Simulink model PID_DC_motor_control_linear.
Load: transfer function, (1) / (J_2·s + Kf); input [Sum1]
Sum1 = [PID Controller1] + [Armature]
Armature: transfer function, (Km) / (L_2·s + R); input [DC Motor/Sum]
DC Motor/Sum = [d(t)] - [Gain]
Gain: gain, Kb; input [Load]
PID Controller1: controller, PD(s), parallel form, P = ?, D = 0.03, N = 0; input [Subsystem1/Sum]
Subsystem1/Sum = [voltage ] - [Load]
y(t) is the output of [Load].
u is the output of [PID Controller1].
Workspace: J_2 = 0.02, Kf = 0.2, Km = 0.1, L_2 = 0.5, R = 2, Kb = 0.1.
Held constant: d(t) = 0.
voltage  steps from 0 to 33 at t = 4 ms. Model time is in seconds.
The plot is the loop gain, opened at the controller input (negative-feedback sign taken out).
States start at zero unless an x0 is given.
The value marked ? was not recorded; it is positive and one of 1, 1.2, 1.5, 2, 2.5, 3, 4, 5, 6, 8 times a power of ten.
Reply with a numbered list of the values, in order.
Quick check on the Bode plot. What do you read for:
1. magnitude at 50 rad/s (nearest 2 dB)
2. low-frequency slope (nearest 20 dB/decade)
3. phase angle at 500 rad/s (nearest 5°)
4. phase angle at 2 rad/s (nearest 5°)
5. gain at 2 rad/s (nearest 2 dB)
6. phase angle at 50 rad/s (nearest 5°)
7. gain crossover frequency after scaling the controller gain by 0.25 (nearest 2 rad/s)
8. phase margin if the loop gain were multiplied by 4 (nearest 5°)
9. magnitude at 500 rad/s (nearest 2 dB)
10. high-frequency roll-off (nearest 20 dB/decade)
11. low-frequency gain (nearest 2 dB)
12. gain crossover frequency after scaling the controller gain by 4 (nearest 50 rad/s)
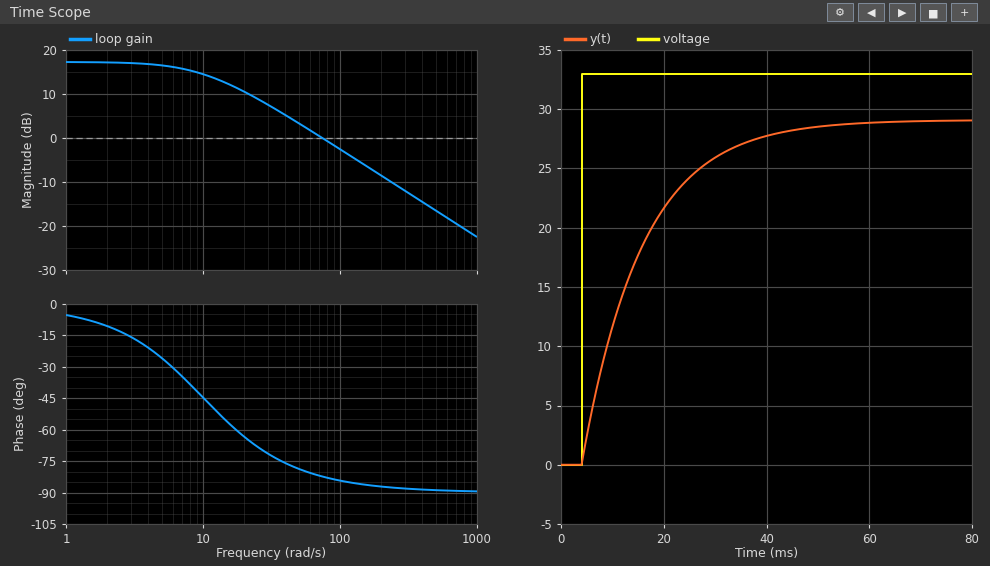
1. 4 dB
2. 0 dB/decade
3. -90°
4. -10°
5. 18 dB
6. -80°
7. 16 rad/s
8. 90°
9. -16 dB
10. -20 dB/decade
11. 18 dB
12. 300 rad/s
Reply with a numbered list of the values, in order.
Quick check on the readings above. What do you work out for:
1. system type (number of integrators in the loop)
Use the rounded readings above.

1. 0
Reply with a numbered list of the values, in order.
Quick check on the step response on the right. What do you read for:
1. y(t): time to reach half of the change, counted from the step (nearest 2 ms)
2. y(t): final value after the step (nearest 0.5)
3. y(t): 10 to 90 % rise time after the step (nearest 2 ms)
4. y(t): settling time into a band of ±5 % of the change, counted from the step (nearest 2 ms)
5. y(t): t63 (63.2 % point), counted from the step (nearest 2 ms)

1. 8 ms
2. 29.0
3. 26 ms
4. 34 ms
5. 12 ms
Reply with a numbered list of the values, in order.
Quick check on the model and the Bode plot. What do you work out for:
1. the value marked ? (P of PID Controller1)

1. 1.5
